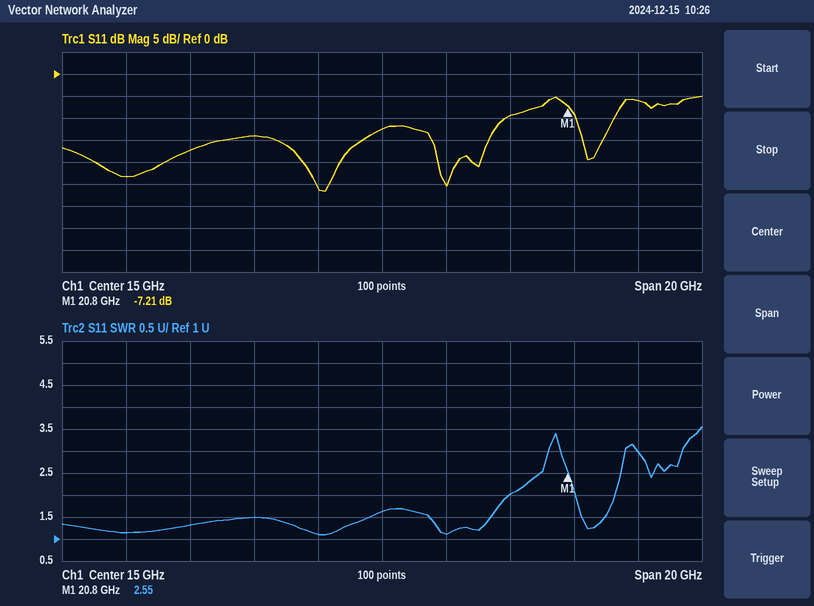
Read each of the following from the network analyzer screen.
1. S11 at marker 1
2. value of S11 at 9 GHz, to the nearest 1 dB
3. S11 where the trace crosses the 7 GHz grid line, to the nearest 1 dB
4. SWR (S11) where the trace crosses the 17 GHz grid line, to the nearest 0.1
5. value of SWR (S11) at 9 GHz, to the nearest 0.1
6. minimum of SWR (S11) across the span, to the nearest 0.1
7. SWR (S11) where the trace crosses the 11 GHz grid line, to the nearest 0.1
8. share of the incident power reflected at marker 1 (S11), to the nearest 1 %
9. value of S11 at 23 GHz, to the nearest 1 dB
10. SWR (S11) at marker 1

-7.21 dB
-17 dB
-23 dB
1.1
1.3
1.1
1.5
19 %
-6 dB
2.55
